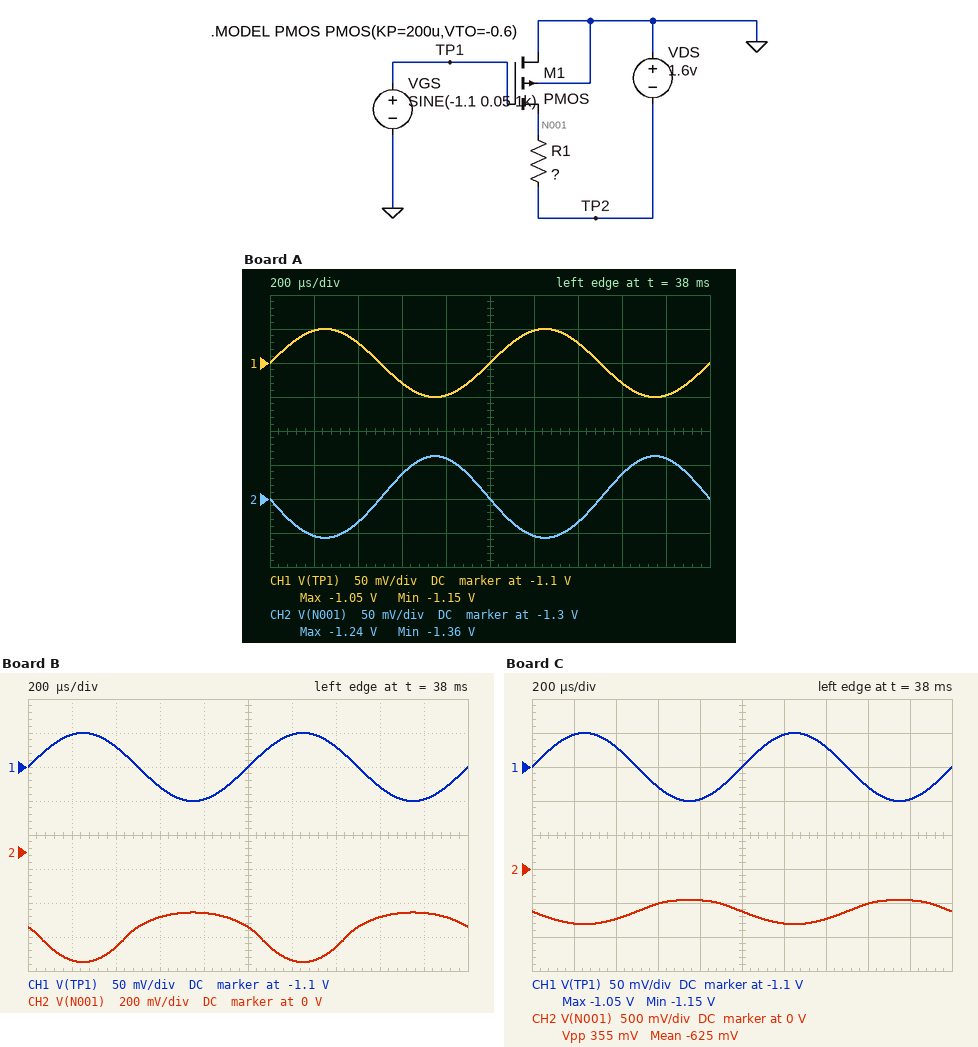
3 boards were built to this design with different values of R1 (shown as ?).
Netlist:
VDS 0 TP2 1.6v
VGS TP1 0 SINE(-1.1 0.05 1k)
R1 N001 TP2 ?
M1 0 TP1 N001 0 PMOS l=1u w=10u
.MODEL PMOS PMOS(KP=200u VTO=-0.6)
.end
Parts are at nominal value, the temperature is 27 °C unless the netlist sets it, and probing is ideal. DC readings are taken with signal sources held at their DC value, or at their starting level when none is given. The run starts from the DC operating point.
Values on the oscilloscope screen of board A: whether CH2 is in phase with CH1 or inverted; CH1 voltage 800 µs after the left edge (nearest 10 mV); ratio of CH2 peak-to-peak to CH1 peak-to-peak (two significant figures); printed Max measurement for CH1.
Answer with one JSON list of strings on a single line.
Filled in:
["inverted", "-1.15 V", "1.2", "-1.05 V"]
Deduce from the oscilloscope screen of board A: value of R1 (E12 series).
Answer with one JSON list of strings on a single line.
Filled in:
["1.2 kΩ"]
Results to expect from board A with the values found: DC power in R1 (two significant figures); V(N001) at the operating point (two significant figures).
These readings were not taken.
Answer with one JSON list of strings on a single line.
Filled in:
["75 µW", "-1.3 V"]
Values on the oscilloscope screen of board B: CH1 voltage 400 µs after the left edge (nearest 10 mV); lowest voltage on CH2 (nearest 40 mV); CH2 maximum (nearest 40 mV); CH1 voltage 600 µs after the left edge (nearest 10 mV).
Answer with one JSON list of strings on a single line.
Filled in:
["-1.07 V", "-640 mV", "-360 mV", "-1.13 V"]
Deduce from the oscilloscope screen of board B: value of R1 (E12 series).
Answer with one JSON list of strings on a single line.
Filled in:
["4.7 kΩ"]
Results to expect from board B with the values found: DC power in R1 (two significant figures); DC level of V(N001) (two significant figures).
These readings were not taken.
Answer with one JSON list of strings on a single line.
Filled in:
["290 µW", "-440 mV"]
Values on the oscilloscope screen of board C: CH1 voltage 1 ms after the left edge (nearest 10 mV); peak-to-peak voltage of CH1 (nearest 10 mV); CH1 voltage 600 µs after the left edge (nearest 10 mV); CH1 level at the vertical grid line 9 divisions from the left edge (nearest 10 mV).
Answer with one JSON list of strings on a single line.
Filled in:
["-1.10 V", "100 mV", "-1.13 V", "-1.15 V"]
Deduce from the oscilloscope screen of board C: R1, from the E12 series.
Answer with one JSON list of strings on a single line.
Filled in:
["3.9 kΩ"]
